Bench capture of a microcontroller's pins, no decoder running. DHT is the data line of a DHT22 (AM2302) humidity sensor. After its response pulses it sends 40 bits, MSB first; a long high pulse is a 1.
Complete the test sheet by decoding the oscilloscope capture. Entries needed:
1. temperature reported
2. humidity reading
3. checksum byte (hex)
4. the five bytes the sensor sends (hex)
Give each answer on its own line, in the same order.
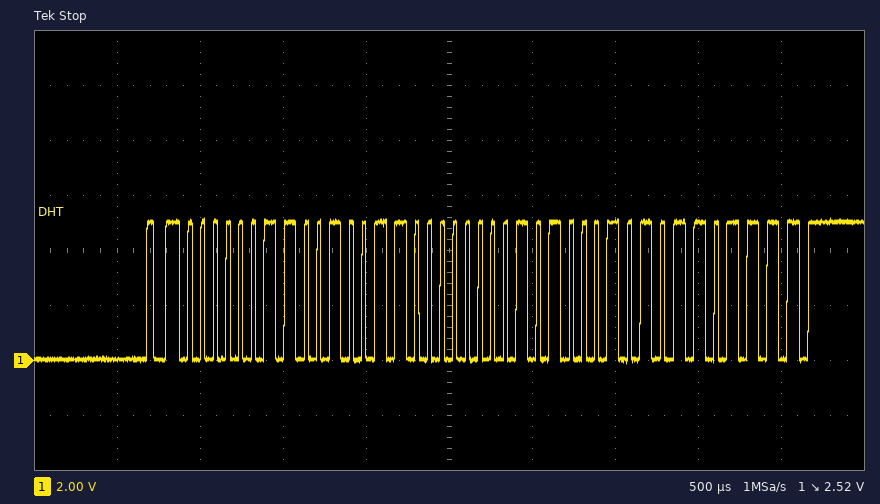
32.5 °C
80.6 %
0x6F
03 26 01 45 6F
